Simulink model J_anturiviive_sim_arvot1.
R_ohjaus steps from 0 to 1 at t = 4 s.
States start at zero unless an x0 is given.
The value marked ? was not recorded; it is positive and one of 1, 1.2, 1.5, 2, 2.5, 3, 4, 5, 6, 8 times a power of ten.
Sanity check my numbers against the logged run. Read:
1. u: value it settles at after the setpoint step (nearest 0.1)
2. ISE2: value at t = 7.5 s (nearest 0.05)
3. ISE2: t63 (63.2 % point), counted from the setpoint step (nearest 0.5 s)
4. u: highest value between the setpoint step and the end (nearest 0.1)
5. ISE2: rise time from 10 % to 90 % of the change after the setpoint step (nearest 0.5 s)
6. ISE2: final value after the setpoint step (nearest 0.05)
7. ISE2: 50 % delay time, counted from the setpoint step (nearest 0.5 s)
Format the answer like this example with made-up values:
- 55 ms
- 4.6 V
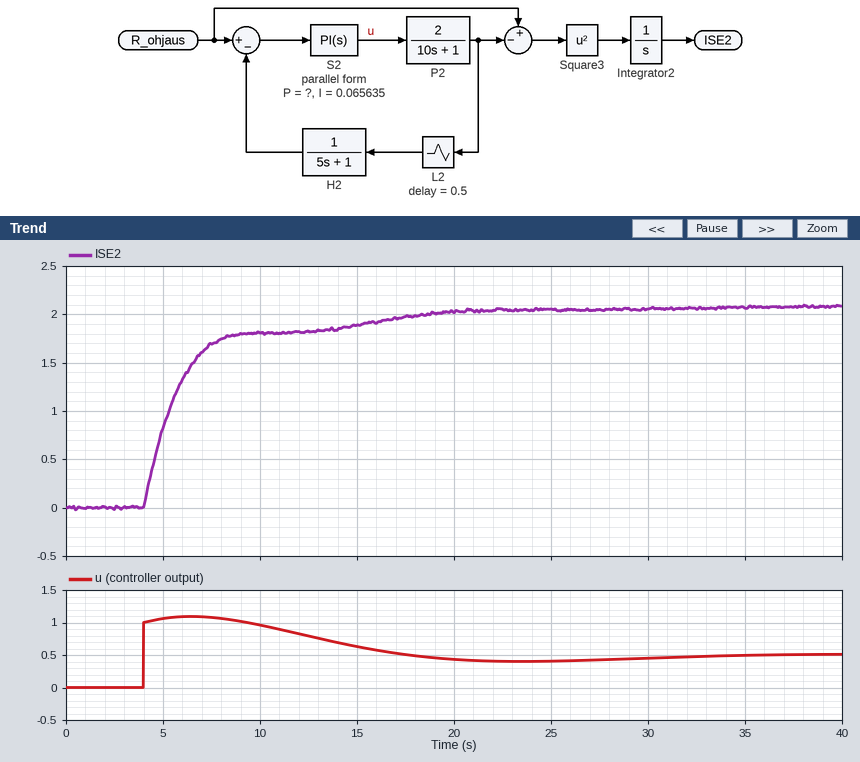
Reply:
- 0.5
- 1.70
- 2.0 s
- 1.1
- 10.5 s
- 2.10
- 1.5 s
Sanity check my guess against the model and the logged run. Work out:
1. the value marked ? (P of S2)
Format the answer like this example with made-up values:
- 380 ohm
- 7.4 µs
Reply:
- 1
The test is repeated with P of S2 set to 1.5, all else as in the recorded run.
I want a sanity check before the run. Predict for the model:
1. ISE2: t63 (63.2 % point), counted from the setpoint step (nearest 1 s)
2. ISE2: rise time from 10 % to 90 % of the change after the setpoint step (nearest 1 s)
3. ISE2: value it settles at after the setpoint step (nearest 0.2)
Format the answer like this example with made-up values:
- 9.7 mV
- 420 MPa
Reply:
- 6 s
- 13 s
- 2.0
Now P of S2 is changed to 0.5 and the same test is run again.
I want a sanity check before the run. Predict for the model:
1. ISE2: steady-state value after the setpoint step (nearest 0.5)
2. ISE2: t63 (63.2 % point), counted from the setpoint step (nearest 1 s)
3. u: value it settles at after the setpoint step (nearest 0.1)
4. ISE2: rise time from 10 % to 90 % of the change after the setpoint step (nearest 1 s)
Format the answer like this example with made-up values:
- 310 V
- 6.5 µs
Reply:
- 4.0
- 4 s
- 0.5
- 19 s
